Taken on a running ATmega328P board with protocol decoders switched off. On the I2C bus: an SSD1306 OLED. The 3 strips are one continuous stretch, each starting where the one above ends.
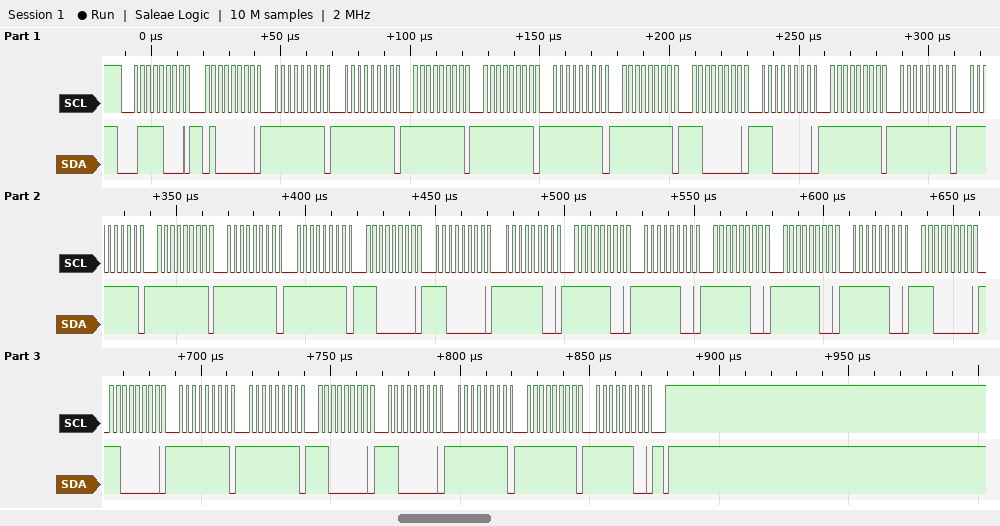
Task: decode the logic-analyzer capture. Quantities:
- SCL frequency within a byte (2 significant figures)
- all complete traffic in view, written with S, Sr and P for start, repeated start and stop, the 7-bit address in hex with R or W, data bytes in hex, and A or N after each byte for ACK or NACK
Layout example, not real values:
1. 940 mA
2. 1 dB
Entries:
1. 400 kHz
2. S 3CW A 40 A FF A FF A FF A FF A FF A FF A C0 A C0 A FF A FF A FF A FF A FF A FF A C0 A C0 A FC A FC A FC A FC A FC A FC A C0 A C0 A FF A FF A C0 A C0 A FF A FF A FC A P
